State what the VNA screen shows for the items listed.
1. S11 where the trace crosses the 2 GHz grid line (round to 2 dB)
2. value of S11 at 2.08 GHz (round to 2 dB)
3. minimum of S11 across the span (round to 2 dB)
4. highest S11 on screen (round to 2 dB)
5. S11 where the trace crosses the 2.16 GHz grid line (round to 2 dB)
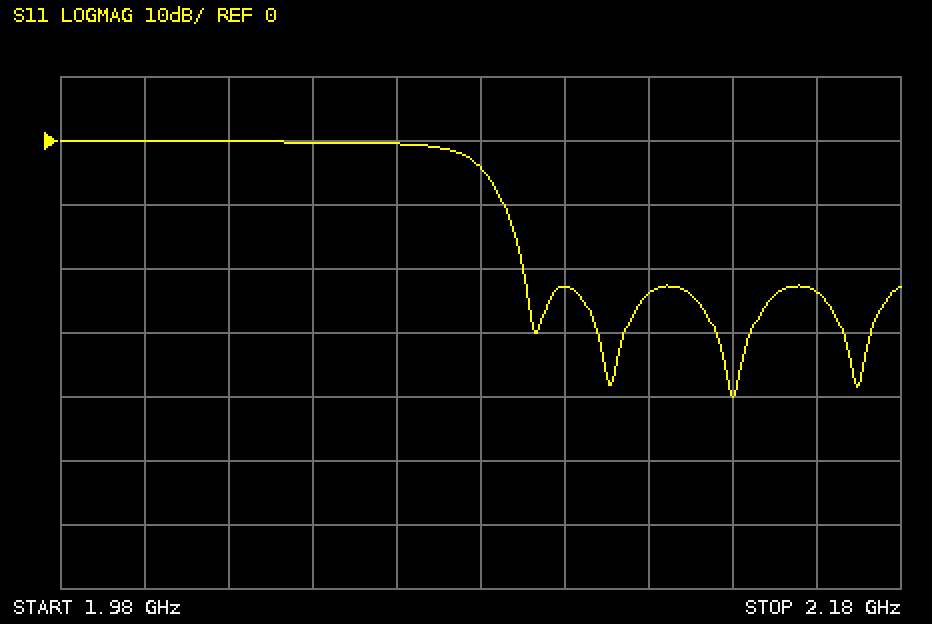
0 dB
-4 dB
-40 dB
0 dB
-24 dB
